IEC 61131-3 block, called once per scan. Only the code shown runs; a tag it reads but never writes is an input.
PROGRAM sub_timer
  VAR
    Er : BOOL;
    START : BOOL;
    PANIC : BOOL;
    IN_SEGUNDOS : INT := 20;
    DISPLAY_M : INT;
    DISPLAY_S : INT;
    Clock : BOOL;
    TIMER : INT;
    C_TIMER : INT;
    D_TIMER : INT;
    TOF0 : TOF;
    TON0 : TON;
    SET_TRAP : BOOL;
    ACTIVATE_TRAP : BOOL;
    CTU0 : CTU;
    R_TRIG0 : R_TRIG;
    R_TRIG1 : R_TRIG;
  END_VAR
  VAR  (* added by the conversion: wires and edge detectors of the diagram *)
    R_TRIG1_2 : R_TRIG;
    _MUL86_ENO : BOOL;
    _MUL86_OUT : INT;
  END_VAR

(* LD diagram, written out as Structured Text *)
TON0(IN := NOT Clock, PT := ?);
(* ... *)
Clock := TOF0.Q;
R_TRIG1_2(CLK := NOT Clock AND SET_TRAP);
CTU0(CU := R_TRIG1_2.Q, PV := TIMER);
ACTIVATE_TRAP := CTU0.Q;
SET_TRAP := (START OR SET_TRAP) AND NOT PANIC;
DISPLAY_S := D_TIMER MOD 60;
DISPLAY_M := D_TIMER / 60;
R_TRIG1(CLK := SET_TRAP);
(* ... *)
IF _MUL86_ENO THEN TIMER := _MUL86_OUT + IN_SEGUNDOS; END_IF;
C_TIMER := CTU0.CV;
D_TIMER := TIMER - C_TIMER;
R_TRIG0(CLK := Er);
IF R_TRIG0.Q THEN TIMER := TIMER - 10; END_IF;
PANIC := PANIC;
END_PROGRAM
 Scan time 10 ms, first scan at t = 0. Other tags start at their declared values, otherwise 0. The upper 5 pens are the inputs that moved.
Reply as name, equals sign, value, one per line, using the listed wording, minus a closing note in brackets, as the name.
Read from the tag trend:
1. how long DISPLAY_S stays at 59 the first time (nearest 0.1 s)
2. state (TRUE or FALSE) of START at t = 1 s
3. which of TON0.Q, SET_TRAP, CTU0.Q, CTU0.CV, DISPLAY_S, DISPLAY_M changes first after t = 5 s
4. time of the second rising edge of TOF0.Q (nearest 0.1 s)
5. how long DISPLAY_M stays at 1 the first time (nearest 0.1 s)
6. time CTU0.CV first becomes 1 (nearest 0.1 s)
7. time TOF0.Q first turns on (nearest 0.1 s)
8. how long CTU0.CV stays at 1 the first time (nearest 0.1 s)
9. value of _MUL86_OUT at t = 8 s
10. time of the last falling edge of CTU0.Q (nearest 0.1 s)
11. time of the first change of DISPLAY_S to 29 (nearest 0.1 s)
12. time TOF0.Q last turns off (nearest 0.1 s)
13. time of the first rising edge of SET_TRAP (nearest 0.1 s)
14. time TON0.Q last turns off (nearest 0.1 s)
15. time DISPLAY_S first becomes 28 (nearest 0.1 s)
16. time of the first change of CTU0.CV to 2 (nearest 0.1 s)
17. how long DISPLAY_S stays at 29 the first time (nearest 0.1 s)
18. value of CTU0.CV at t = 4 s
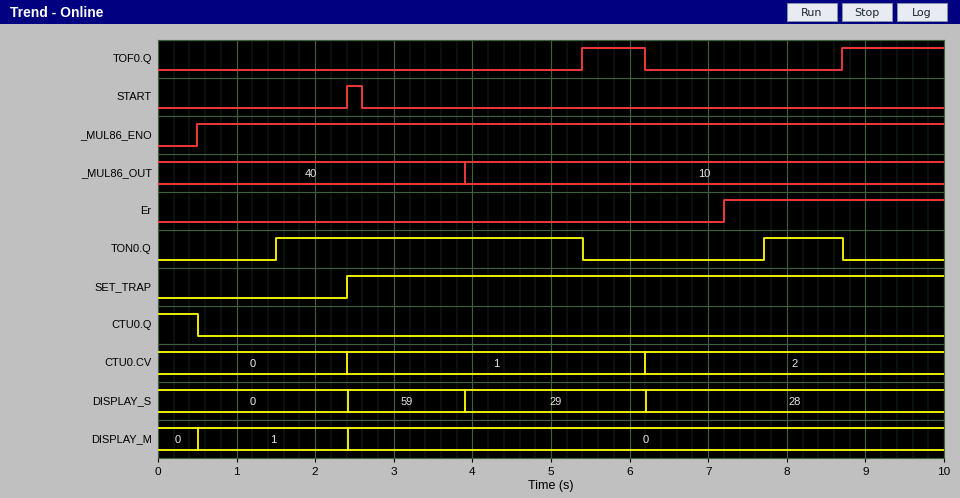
how long DISPLAY_S stays at 59 the first time = 1.5 s
state (TRUE or FALSE) of START at t = 1 s = FALSE
which of TON0.Q, SET_TRAP, CTU0.Q, CTU0.CV, DISPLAY_S, DISPLAY_M changes first after t = 5 s = TON0.Q
time of the second rising edge of TOF0.Q = 8.7 s
how long DISPLAY_M stays at 1 the first time = 1.9 s
time CTU0.CV first becomes 1 = 2.4 s
time TOF0.Q first turns on = 5.4 s
how long CTU0.CV stays at 1 the first time = 3.8 s
value of _MUL86_OUT at t = 8 s = 10
time of the last falling edge of CTU0.Q = 0.5 s
time of the first change of DISPLAY_S to 29 = 3.9 s
time TOF0.Q last turns off = 6.2 s
time of the first rising edge of SET_TRAP = 2.4 s
time TON0.Q last turns off = 8.7 s
time DISPLAY_S first becomes 28 = 6.2 s
time of the first change of CTU0.CV to 2 = 6.2 s
how long DISPLAY_S stays at 29 the first time = 2.3 s
value of CTU0.CV at t = 4 s = 1
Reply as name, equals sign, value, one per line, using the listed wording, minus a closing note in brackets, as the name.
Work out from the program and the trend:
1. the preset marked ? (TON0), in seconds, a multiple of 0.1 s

the preset marked ? (TON0), in seconds, a multiple of 0.1 s = 1.5 s
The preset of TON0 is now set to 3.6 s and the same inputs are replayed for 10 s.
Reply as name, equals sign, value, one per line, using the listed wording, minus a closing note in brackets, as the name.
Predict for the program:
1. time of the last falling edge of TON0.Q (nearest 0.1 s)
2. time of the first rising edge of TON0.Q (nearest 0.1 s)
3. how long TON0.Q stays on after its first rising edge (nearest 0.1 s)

time of the last falling edge of TON0.Q = 5.4 s
time of the first rising edge of TON0.Q = 3.6 s
how long TON0.Q stays on after its first rising edge = 1.8 s
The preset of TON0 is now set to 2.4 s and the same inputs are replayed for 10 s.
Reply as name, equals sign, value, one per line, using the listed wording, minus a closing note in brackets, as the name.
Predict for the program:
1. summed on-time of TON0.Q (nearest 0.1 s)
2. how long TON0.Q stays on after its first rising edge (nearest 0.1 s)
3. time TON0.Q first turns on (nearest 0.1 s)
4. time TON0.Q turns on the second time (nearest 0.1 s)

summed on-time of TON0.Q = 3.1 s
how long TON0.Q stays on after its first rising edge = 3.0 s
time TON0.Q first turns on = 2.4 s
time TON0.Q turns on the second time = 8.6 s
